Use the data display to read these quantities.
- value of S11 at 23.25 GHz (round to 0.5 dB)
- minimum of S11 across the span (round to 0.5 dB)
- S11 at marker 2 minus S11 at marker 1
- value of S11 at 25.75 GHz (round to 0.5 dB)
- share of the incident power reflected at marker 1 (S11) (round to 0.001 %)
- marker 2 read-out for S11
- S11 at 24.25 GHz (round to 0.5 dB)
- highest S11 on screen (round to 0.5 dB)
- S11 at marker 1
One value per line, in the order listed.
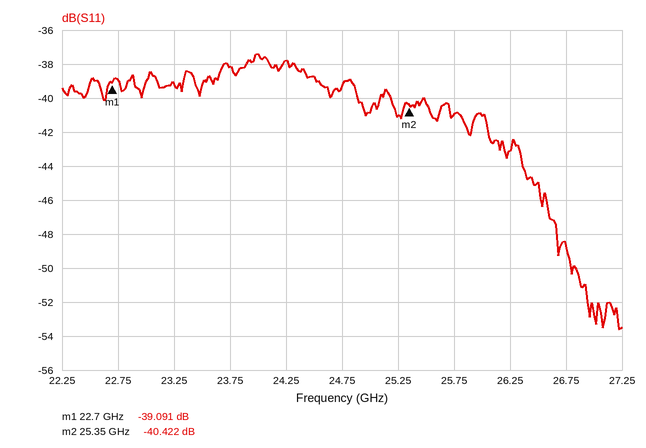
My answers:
-39.0 dB
-53.5 dB
-1.331 dB
-41.0 dB
0.012 %
-40.422 dB
-38.0 dB
-37.5 dB
-39.091 dB
